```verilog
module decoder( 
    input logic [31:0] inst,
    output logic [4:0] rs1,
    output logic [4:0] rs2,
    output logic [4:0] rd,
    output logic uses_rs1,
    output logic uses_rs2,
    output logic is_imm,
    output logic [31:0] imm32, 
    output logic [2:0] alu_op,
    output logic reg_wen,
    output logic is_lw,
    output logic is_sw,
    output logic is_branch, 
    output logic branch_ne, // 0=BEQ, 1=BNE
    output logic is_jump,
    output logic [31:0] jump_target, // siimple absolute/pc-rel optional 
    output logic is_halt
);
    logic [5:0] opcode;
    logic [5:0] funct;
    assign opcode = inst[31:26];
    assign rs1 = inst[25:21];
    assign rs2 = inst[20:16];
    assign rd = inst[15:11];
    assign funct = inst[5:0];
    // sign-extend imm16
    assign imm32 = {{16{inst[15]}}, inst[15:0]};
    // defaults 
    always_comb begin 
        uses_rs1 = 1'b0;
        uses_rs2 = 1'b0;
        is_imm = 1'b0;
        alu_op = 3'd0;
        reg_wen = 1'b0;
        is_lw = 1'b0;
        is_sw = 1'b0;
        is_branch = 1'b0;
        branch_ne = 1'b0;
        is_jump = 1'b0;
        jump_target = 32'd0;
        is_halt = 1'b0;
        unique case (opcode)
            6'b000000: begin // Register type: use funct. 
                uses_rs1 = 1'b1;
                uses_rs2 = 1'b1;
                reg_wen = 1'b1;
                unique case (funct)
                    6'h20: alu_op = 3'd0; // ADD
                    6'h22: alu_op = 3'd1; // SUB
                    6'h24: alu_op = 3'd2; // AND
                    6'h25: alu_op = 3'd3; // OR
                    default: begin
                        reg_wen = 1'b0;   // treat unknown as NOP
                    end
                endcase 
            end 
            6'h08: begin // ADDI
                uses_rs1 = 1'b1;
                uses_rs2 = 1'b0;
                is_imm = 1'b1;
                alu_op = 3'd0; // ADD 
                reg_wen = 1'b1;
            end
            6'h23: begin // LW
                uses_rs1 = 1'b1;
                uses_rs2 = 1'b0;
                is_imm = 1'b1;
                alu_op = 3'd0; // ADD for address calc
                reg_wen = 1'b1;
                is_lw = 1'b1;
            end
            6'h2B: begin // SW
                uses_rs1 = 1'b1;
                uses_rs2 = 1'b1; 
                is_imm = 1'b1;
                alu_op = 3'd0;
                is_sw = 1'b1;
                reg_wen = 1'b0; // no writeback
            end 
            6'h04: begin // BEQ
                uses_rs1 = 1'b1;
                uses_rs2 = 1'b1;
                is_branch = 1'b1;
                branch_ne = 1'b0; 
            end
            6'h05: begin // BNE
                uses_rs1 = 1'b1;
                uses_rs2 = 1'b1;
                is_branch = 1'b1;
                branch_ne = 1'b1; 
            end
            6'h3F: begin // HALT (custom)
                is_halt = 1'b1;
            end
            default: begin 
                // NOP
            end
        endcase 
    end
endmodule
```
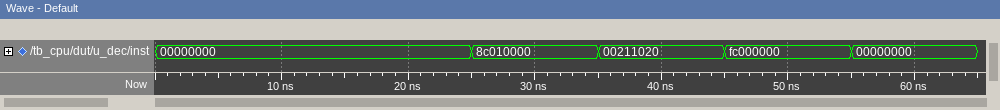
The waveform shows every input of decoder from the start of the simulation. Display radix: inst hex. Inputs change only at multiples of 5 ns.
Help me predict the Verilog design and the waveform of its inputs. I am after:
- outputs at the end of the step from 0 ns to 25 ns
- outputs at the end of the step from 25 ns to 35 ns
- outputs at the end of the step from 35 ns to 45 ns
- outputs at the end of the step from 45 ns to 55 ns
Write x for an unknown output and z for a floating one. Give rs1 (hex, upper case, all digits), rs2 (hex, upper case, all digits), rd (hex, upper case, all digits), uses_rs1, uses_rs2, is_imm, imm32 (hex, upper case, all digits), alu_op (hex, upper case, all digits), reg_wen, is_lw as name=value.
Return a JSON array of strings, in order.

["rs1=00, rs2=00, rd=00, uses_rs1=1, uses_rs2=1, is_imm=0, imm32=00000000, alu_op=0, reg_wen=0, is_lw=0", "rs1=00, rs2=01, rd=00, uses_rs1=1, uses_rs2=0, is_imm=1, imm32=00000000, alu_op=0, reg_wen=1, is_lw=1", "rs1=01, rs2=01, rd=02, uses_rs1=1, uses_rs2=1, is_imm=0, imm32=00001020, alu_op=0, reg_wen=1, is_lw=0", "rs1=00, rs2=00, rd=00, uses_rs1=0, uses_rs2=0, is_imm=0, imm32=00000000, alu_op=0, reg_wen=0, is_lw=0"]
